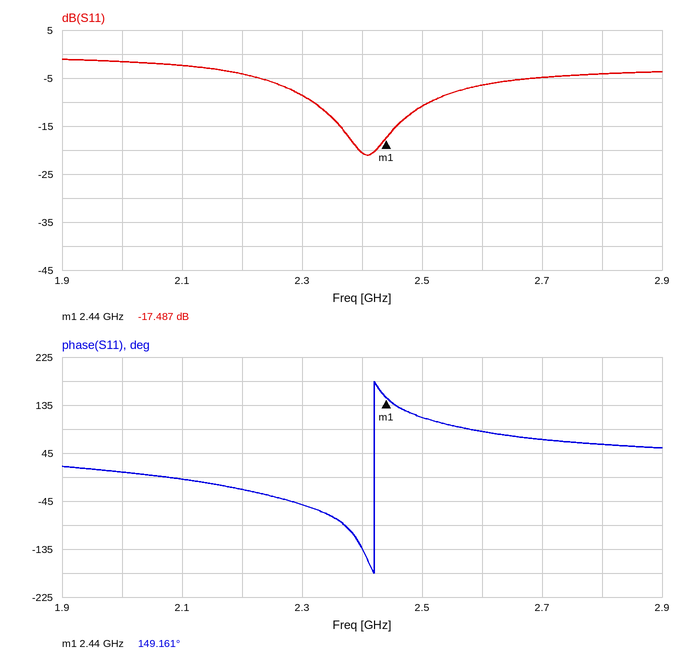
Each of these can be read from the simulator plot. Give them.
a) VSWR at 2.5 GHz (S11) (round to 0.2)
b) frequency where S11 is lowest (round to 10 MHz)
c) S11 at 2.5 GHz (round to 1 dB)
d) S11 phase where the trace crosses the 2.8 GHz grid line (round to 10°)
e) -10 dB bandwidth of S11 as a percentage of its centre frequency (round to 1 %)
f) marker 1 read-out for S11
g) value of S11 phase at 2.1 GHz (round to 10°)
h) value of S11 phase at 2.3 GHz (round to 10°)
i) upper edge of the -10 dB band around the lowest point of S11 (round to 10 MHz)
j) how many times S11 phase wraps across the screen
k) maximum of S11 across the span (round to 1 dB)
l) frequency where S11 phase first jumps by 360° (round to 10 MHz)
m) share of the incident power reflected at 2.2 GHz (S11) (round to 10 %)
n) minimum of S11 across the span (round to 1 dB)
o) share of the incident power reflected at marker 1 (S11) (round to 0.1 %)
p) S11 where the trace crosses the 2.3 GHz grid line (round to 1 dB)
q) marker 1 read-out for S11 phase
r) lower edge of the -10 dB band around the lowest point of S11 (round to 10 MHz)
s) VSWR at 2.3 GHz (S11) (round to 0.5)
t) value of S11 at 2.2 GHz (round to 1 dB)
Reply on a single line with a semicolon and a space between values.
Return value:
1.8; 2.41 GHz; -11 dB; 60°; 8 %; -17.487 dB; 0°; -50°; 2.51 GHz; 1; -1 dB; 2.42 GHz; 40 %; -21 dB; 1.8 %; -9 dB; 149.161°; 2.32 GHz; 2.0; -4 dB
